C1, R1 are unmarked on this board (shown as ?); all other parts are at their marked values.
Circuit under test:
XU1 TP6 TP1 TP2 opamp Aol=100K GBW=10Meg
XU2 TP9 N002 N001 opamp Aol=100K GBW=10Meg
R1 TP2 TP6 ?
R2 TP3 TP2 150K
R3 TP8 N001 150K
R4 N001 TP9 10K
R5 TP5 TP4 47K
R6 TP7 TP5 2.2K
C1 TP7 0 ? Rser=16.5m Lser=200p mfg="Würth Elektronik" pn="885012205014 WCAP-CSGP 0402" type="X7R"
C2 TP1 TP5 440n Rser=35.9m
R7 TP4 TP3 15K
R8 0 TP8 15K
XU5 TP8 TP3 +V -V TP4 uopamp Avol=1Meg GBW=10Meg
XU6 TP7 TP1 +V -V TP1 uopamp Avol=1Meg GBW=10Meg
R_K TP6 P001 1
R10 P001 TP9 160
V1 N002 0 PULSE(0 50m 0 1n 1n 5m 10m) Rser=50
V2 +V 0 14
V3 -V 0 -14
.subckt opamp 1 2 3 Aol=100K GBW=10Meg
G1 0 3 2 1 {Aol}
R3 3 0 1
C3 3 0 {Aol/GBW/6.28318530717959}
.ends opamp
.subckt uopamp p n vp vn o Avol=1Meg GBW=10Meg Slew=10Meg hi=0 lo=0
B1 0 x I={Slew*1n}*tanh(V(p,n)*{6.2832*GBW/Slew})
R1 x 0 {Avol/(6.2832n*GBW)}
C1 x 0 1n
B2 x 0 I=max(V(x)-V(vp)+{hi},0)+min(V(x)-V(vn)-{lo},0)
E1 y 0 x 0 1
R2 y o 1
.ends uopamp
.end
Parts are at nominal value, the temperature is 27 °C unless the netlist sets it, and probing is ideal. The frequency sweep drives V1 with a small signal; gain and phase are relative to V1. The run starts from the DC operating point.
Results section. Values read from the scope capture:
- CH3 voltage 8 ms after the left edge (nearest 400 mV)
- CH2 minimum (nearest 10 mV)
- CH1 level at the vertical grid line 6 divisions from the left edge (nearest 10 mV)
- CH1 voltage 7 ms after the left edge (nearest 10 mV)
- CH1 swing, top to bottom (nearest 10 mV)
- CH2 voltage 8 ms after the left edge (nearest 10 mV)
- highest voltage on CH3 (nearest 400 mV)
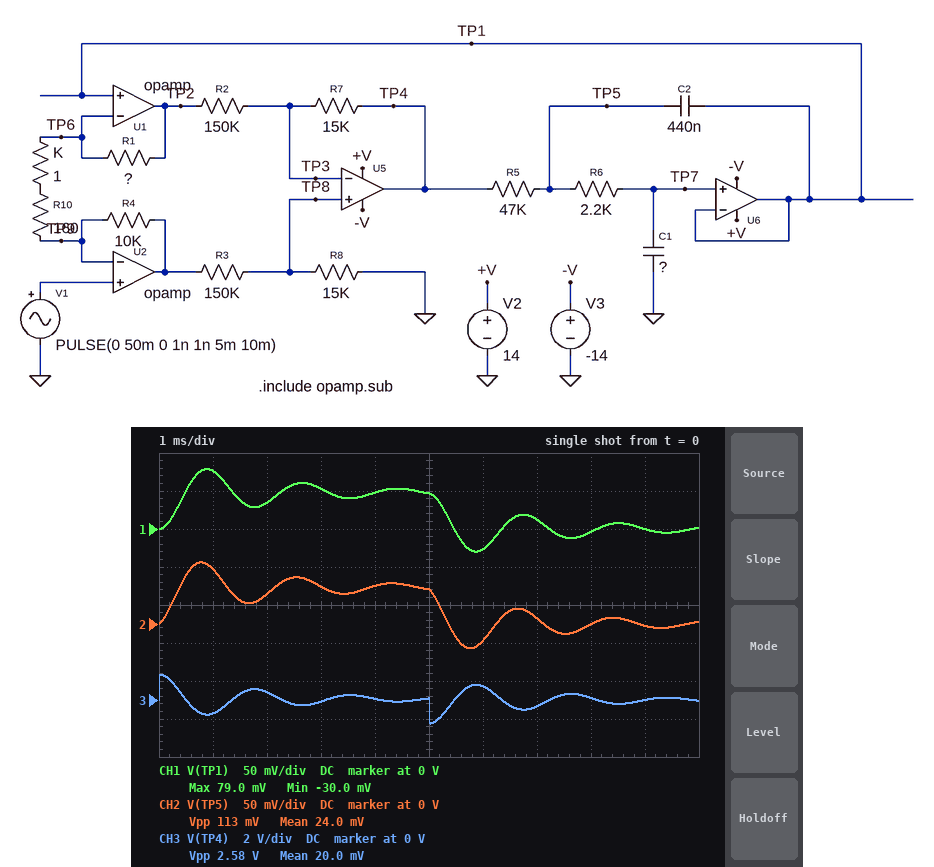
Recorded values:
0 V
-30 mV
-30 mV
10 mV
110 mV
0 V
1.2 V
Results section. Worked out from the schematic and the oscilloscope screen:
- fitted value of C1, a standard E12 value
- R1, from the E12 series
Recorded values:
47 nF
33 kΩ
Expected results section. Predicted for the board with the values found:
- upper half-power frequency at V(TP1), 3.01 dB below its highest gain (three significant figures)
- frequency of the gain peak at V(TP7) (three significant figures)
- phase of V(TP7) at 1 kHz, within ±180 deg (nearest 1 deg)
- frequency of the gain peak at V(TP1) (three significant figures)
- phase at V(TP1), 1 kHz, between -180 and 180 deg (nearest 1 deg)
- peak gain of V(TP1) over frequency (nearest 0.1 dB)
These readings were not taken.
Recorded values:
639 Hz
561 Hz
-168 deg
561 Hz
-168 deg
10.7 dB
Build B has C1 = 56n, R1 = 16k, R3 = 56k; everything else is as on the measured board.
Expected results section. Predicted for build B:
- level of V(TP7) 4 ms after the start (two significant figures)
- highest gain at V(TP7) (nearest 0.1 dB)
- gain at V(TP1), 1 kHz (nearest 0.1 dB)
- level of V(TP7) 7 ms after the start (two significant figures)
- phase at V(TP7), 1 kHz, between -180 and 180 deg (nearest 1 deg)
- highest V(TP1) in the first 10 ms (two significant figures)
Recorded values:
43 mV
9.3 dB
-9.9 dB
18 mV
-168 deg
77 mV
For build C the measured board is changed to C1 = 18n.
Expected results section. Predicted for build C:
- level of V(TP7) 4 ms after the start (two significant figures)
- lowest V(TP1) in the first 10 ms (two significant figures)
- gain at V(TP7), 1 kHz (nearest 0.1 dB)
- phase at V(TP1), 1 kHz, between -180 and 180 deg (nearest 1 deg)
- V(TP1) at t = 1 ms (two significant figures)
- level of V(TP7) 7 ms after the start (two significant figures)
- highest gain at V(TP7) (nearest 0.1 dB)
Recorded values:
52 mV
-40 mV
12.0 dB
-135 deg
23 mV
11 mV
15.5 dB
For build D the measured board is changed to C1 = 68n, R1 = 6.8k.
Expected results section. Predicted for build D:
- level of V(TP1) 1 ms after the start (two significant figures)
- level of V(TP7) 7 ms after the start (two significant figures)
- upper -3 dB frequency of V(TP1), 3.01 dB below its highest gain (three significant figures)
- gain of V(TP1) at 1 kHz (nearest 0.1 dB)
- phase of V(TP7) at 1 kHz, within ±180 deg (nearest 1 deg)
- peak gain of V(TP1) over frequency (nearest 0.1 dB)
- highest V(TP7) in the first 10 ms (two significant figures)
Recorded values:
46 mV
-17 mV
361 Hz
-20.6 dB
-170 deg
4.6 dB
64 mV
